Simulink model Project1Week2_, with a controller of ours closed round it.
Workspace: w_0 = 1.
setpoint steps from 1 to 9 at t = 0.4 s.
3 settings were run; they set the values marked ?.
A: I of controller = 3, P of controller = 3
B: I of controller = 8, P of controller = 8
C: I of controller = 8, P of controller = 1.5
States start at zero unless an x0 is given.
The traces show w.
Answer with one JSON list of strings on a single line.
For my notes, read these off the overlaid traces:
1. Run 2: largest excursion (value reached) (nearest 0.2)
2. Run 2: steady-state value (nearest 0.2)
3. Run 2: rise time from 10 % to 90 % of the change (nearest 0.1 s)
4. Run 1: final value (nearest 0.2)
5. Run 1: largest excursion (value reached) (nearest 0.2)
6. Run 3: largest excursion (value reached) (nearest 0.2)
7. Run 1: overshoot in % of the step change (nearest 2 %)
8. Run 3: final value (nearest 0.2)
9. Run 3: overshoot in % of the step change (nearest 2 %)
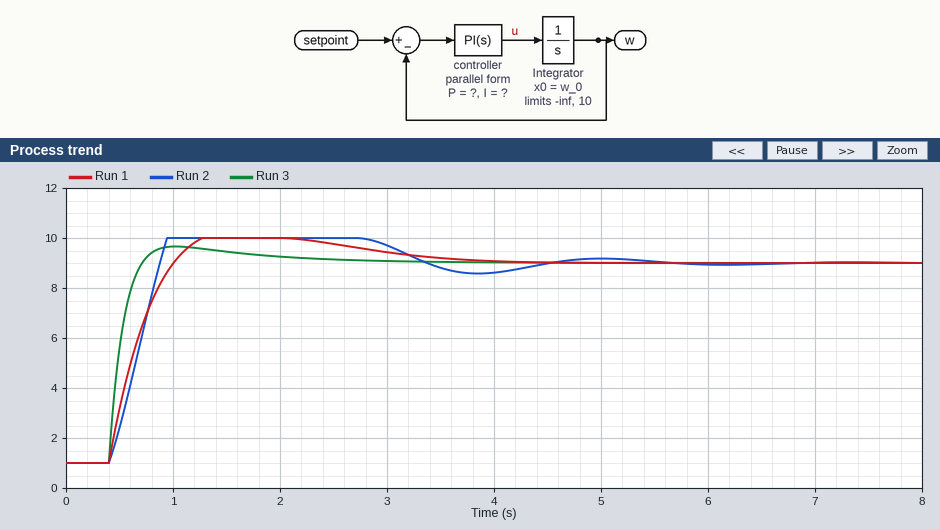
["10.0", "9.0", "0.4 s", "9.0", "10.0", "9.6", "12 %", "9.0", "8 %"]
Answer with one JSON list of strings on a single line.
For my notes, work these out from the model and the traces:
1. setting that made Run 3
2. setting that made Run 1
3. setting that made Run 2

["B", "A", "C"]
